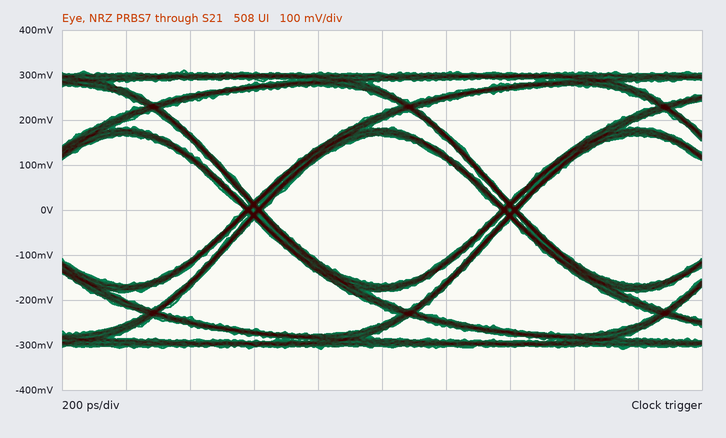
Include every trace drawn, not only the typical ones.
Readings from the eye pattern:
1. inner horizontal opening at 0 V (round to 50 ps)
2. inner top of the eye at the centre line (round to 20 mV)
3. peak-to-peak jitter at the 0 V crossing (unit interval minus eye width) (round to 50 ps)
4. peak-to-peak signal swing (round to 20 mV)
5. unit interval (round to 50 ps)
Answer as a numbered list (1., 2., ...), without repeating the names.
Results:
1. 750 ps
2. 160 mV
3. 50 ps
4. 620 mV
5. 800 ps
